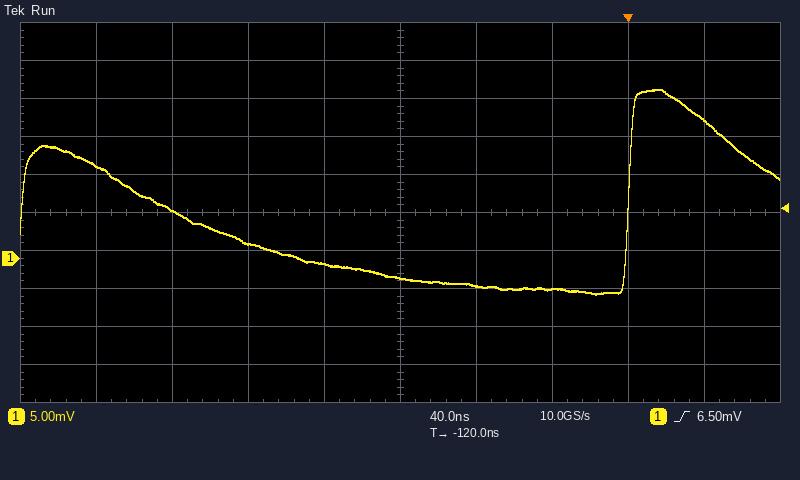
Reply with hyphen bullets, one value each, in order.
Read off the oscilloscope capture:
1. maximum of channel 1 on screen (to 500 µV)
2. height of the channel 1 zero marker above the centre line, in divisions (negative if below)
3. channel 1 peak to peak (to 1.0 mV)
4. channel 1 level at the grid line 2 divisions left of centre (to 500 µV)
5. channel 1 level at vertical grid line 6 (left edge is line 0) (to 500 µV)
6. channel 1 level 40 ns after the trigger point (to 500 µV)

- 22.0 mV
- -1.2 div
- 27.0 mV
- 2.0 mV
- -3.5 mV
- 18.0 mV
